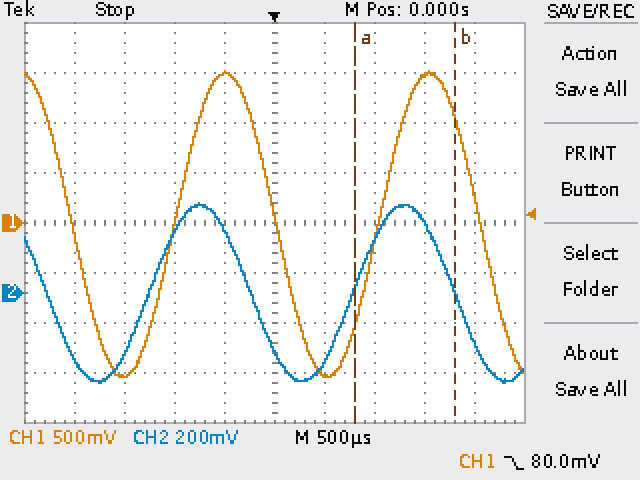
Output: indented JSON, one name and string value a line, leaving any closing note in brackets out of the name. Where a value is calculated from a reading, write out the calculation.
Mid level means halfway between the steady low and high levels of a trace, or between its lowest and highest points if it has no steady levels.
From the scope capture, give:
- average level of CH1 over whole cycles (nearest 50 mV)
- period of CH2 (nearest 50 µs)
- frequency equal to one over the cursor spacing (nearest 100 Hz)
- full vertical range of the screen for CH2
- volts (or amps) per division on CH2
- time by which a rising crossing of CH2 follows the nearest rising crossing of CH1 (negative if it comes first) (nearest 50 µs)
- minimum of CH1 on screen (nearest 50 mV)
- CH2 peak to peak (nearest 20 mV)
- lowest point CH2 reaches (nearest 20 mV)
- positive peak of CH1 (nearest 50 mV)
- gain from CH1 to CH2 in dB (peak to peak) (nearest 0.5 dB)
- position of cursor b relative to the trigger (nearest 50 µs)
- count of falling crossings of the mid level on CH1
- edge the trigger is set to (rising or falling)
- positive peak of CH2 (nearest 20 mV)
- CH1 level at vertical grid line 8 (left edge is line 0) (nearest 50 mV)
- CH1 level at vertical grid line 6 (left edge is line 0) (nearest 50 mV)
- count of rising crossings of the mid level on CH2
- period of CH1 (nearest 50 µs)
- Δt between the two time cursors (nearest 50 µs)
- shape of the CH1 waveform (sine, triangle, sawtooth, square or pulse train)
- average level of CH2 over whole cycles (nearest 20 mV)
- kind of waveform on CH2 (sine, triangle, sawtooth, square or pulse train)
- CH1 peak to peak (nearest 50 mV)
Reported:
{
  "average level of CH1 over whole cycles": "(1.50 V + (-1.55 V)) / 2 ≈ 0 mV",
  "period of CH2": "2.05 ms",
  "frequency equal to one over the cursor spacing": "1 / 1.00 ms ≈ 1.0 kHz",
  "full vertical range of the screen for CH2": "1.6 V",
  "volts (or amps) per division on CH2": "200 mV",
  "time by which a rising crossing of CH2 follows the nearest rising crossing of CH1 (negative if it comes first)": "-250 µs",
  "minimum of CH1 on screen": "-1.55 V",
  "CH2 peak to peak": "360 mV − (-360 mV) = 720 mV",
  "lowest point CH2 reaches": "-360 mV",
  "positive peak of CH1": "1.50 V",
  "gain from CH1 to CH2 in dB (peak to peak)": "20 log10(720 mV / 3.05 V) ≈ -12.5 dB",
  "position of cursor b relative to the trigger": "+1.80 ms",
  "count of falling crossings of the mid level on CH1": "3",
  "edge the trigger is set to": "falling",
  "positive peak of CH2": "360 mV",
  "CH1 level at vertical grid line 8 (left edge is line 0)": "1.45 V",
  "CH1 level at vertical grid line 6 (left edge is line 0)": "-1.50 V",
  "count of rising crossings of the mid level on CH2": "2",
  "period of CH1": "2.05 ms",
  "Δt between the two time cursors": "1.00 ms",
  "shape of the CH1 waveform": "sine",
  "average level of CH2 over whole cycles": "(360 mV + (-360 mV)) / 2 ≈ 0 mV",
  "kind of waveform on CH2": "sine",
  "CH1 peak to peak": "1.50 V − (-1.55 V) = 3.05 V"
}
